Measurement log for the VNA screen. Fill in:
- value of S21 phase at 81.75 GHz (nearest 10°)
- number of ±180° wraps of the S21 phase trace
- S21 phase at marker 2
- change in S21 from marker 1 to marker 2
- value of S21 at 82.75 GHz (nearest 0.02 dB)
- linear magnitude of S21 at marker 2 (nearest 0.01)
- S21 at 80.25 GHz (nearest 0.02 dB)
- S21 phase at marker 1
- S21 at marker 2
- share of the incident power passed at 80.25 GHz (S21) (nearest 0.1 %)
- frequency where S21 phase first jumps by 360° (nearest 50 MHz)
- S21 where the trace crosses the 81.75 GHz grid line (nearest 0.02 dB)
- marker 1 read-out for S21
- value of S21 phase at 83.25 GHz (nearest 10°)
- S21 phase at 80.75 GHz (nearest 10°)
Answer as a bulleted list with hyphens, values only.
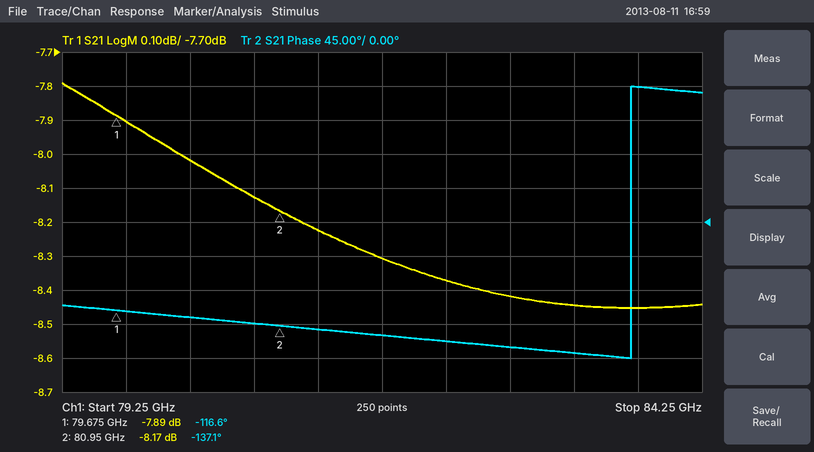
- -150°
- 1
- -137.1°
- -0.28 dB
- -8.42 dB
- 0.39
- -8.02 dB
- -116.6°
- -8.17 dB
- 15.8 %
- 83.70 GHz
- -8.30 dB
- -7.89 dB
- -170°
- -130°
